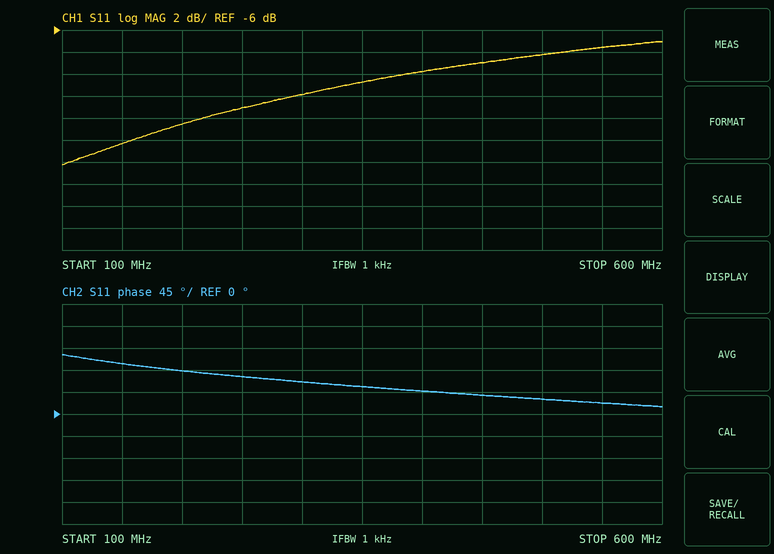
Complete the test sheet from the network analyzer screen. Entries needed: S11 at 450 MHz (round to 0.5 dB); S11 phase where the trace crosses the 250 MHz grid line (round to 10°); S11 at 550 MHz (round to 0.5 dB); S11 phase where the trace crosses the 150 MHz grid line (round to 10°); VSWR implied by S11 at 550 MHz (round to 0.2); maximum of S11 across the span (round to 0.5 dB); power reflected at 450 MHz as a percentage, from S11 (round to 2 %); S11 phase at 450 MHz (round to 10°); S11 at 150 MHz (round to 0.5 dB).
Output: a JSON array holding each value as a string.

["-9.0 dB", "80°", "-7.5 dB", "100°", "2.4", "-7.0 dB", "12 %", "40°", "-16.5 dB"]
